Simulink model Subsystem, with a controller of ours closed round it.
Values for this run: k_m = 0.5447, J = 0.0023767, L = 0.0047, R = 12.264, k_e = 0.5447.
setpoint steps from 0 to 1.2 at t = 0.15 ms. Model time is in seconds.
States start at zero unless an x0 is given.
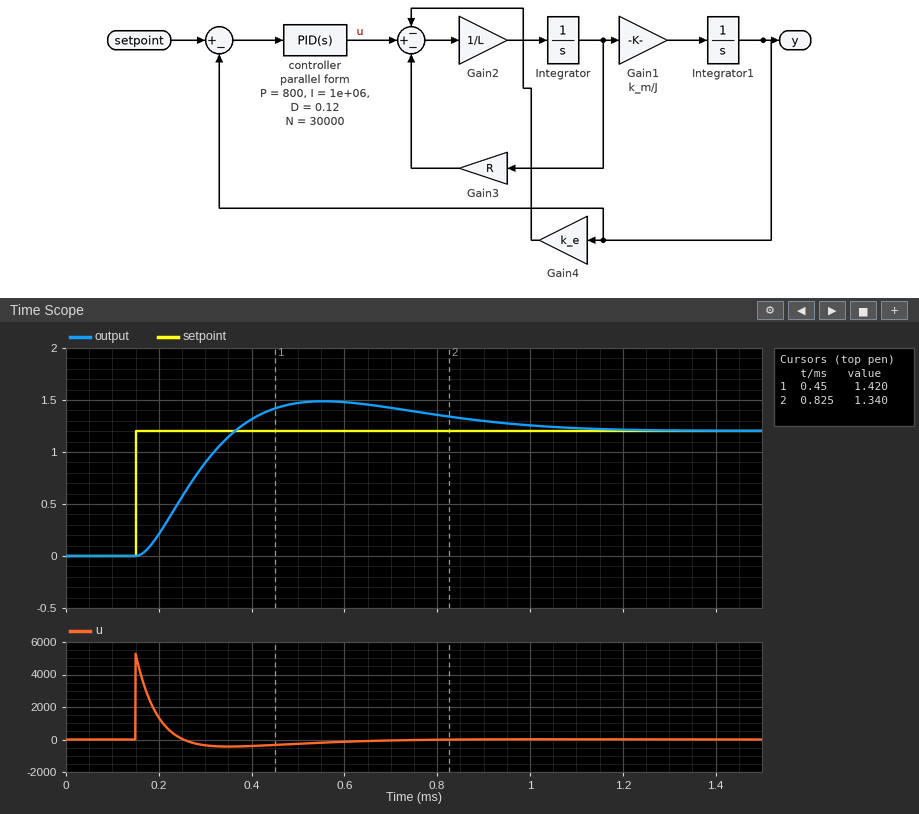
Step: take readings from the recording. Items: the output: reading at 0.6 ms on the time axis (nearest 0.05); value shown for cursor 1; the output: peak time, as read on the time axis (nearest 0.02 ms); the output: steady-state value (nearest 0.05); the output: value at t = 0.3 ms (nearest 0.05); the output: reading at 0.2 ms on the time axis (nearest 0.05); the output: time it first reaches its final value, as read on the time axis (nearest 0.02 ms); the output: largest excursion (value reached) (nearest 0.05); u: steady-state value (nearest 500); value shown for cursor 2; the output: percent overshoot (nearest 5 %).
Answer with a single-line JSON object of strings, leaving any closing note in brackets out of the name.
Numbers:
{"the output: reading at 0.6 ms on the time axis": "1.50", "value shown for cursor 1": "1.420", "the output: peak time, as read on the time axis": "0.56 ms", "the output: steady-state value": "1.20", "the output: value at t = 0.3 ms": "0.90", "the output: reading at 0.2 ms on the time axis": "0.20", "the output: time it first reaches its final value, as read on the time axis": "0.36 ms", "the output: largest excursion (value reached)": "1.50", "u: steady-state value": "0", "value shown for cursor 2": "1.340", "the output: percent overshoot": "25 %"}
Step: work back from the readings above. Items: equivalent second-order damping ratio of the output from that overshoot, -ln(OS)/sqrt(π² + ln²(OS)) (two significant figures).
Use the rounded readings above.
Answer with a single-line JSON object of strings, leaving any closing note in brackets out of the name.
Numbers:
{"equivalent second-order damping ratio of the output from that overshoot, -ln(OS)/sqrt(π² + ln²(OS))": "0.40"}
